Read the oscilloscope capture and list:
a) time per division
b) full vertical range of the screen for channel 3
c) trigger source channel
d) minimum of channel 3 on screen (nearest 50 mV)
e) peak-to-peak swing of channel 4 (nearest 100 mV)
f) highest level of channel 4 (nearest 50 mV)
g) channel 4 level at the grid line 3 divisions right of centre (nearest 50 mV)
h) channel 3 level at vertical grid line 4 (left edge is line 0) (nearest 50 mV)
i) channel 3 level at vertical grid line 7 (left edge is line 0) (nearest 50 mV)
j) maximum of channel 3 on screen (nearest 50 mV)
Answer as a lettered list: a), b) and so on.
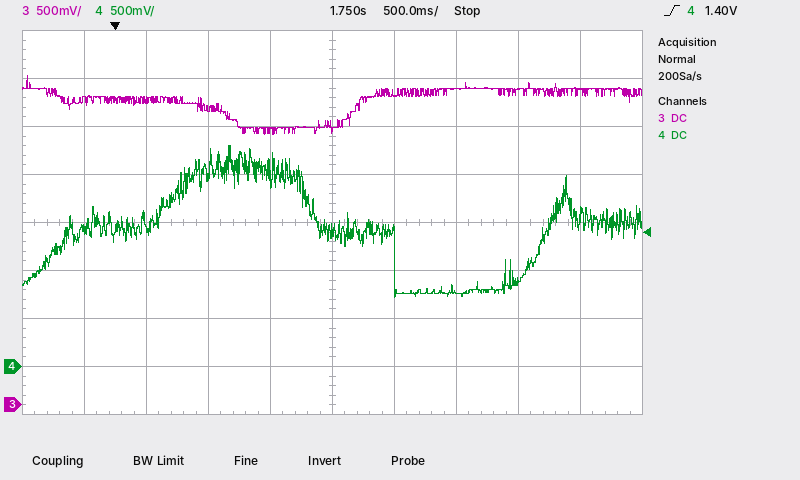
a) 500 ms
b) 4 V
c) channel 4
d) 2.80 V
e) 1.60 V
f) 2.30 V
g) 900 mV
h) 2.85 V
i) 3.30 V
j) 3.45 V
